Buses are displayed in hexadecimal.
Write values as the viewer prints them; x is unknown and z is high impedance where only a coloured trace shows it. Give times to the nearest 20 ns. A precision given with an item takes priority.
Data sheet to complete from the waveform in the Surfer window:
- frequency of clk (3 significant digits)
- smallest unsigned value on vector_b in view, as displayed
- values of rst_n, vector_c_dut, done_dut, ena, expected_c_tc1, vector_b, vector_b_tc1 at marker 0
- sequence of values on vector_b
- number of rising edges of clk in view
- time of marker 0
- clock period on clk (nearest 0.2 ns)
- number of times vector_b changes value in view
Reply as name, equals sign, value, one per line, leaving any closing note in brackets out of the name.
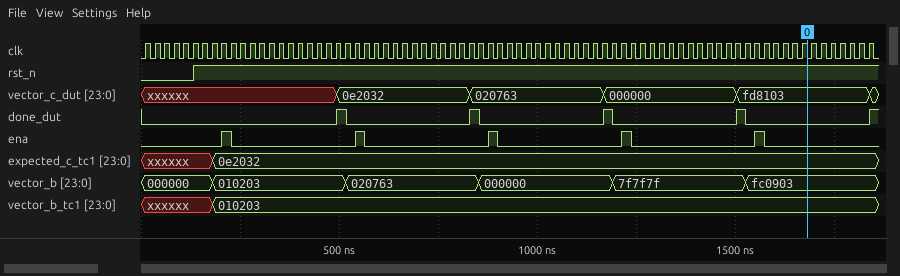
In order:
frequency of clk = 41.7 MHz
smallest unsigned value on vector_b in view, as displayed = 000000
values of rst_n, vector_c_dut, done_dut, ena, expected_c_tc1, vector_b, vector_b_tc1 at marker 0 = rst_n=1, vector_c_dut=fd8103, done_dut=0, ena=0, expected_c_tc1=0e2032, vector_b=fc0903, vector_b_tc1=010203
sequence of values on vector_b = 000000, 010203, 020763, 000000, 7f7f7f, fc0903
number of rising edges of clk in view = 77
time of marker 0 = 1680 ns
clock period on clk = 24 ns
number of times vector_b changes value in view = 5
